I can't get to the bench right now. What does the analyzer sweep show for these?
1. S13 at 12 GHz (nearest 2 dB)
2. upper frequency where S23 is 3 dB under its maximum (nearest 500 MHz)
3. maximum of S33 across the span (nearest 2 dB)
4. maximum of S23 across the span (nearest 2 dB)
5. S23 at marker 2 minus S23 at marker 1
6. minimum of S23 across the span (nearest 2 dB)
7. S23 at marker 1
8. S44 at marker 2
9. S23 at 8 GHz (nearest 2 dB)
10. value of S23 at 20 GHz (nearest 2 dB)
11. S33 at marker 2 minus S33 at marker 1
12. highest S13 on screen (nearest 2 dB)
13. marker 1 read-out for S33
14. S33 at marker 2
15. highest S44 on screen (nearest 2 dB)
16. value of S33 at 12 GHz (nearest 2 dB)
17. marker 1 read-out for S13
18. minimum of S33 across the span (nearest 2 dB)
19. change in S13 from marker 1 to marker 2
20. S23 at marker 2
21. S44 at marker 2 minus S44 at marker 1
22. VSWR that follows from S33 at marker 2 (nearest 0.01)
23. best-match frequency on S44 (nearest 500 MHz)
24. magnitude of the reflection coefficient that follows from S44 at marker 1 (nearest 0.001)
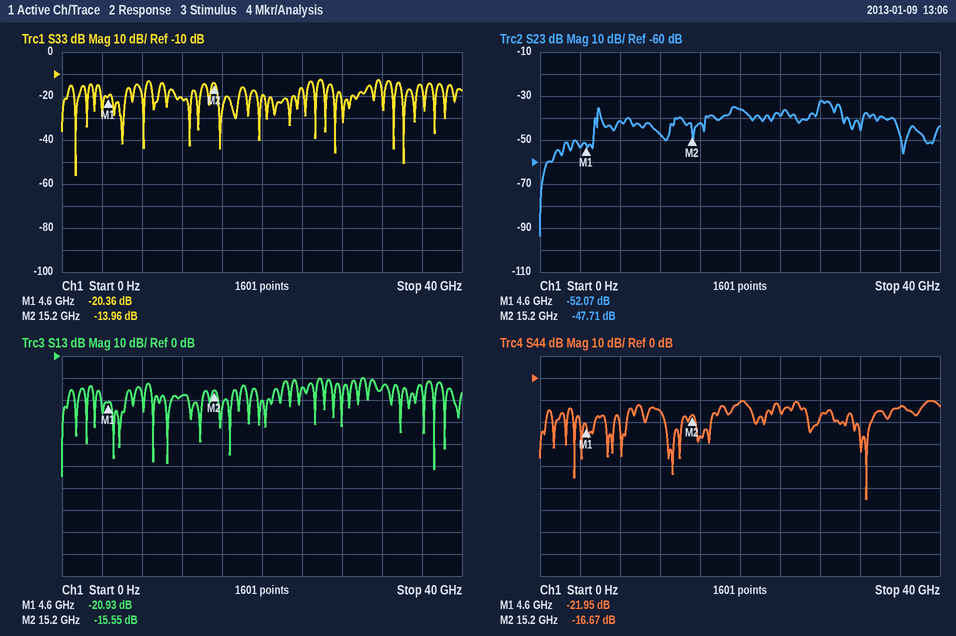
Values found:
-18 dB
29.0 GHz
-12 dB
-32 dB
4.36 dB
-94 dB
-52.07 dB
-16.67 dB
-42 dB
-36 dB
6.40 dB
-10 dB
-20.36 dB
-13.96 dB
-10 dB
-22 dB
-20.93 dB
-56 dB
5.38 dB
-47.71 dB
5.28 dB
1.50
32.5 GHz
0.080
